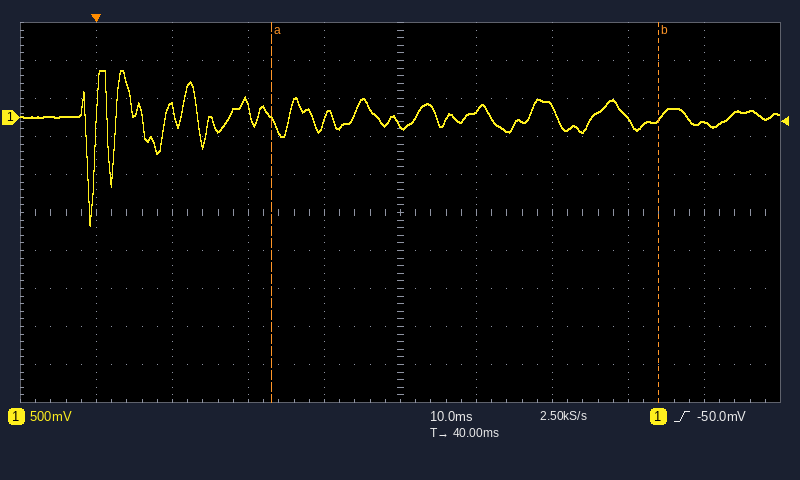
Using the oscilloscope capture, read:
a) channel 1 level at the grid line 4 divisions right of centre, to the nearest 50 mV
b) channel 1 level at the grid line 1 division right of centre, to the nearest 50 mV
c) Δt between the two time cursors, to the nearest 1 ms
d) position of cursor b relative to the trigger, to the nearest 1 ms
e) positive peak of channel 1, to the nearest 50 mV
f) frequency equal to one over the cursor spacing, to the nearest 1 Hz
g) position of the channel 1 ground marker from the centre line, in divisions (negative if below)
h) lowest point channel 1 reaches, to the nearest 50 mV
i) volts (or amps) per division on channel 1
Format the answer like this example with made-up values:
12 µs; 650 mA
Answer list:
-50 mV; 100 mV; 51 ms; +74 ms; 600 mV; 20 Hz; +2.5 div; -1.40 V; 500 mV
